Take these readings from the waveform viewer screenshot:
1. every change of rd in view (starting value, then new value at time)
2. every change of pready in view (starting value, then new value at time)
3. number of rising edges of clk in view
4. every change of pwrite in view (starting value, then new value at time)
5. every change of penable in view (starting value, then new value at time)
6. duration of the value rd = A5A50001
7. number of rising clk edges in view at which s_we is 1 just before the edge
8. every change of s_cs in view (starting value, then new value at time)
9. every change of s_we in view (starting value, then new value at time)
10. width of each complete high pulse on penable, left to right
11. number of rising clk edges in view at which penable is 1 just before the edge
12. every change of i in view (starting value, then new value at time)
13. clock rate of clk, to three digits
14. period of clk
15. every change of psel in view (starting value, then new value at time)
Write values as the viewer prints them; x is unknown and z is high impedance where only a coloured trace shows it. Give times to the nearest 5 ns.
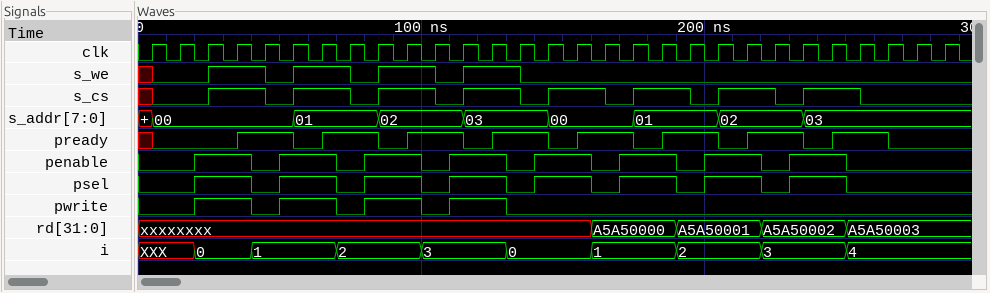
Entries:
xxxxxxxx, A5A50000 at 160 ns, A5A50001 at 190 ns, A5A50002 at 220 ns, A5A50003 at 250 ns
x, 0 at 5 ns, 1 at 35 ns, 0 at 55 ns, 1 at 65 ns, 0 at 85 ns, 1 at 95 ns, 0 at 115 ns, 1 at 125 ns, 0 at 145 ns, 1 at 155 ns, 0 at 175 ns, 1 at 185 ns, 0 at 205 ns, 1 at 215 ns, 0 at 235 ns, 1 at 245 ns, 0 at 265 ns
29
0, 1 at 20 ns, 0 at 40 ns, 1 at 50 ns, 0 at 70 ns, 1 at 80 ns, 0 at 100 ns, 1 at 110 ns, 0 at 130 ns
0, 1 at 20 ns, 0 at 40 ns, 1 at 50 ns, 0 at 70 ns, 1 at 80 ns, 0 at 100 ns, 1 at 110 ns, 0 at 130 ns, 1 at 140 ns, 0 at 160 ns, 1 at 170 ns, 0 at 190 ns, 1 at 200 ns, 0 at 220 ns, 1 at 230 ns, 0 at 250 ns
30 ns
8
x, 0 at 5 ns, 1 at 25 ns, 0 at 45 ns, 1 at 55 ns, 0 at 75 ns, 1 at 85 ns, 0 at 105 ns, 1 at 115 ns, 0 at 135 ns, 1 at 145 ns, 0 at 165 ns, 1 at 175 ns, 0 at 195 ns, 1 at 205 ns, 0 at 225 ns, 1 at 235 ns, 0 at 255 ns
x, 0 at 5 ns, 1 at 25 ns, 0 at 45 ns, 1 at 55 ns, 0 at 75 ns, 1 at 85 ns, 0 at 105 ns, 1 at 115 ns, 0 at 135 ns
20 ns, 20 ns, 20 ns, 20 ns, 20 ns, 20 ns, 20 ns, 20 ns
16
XXX, 0 at 20 ns, 1 at 40 ns, 2 at 70 ns, 3 at 100 ns, 0 at 130 ns, 1 at 160 ns, 2 at 190 ns, 3 at 220 ns, 4 at 250 ns
100 MHz
10 ns
0, 1 at 20 ns, 0 at 40 ns, 1 at 50 ns, 0 at 70 ns, 1 at 80 ns, 0 at 100 ns, 1 at 110 ns, 0 at 130 ns, 1 at 140 ns, 0 at 160 ns, 1 at 170 ns, 0 at 190 ns, 1 at 200 ns, 0 at 220 ns, 1 at 230 ns, 0 at 250 ns
